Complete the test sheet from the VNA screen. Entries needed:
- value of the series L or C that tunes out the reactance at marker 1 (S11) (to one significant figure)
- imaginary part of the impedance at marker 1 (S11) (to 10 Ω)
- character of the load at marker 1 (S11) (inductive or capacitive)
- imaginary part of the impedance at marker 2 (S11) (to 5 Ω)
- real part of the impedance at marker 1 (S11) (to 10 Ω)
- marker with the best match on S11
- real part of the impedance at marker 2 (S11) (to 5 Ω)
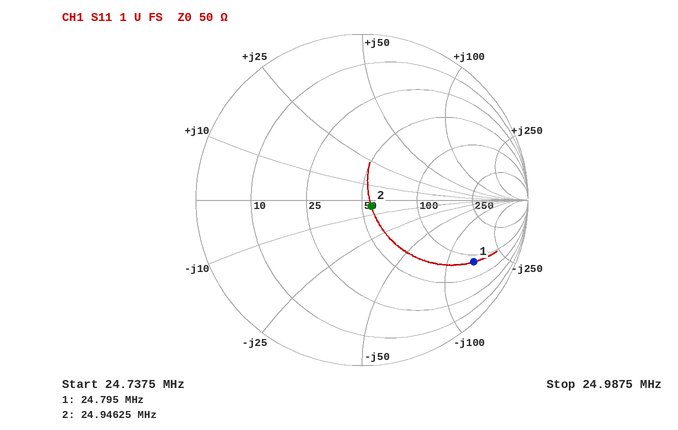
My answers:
1.0 µH
-150 Ω
capacitive
-5 Ω
80 Ω
marker 2
55 Ω
